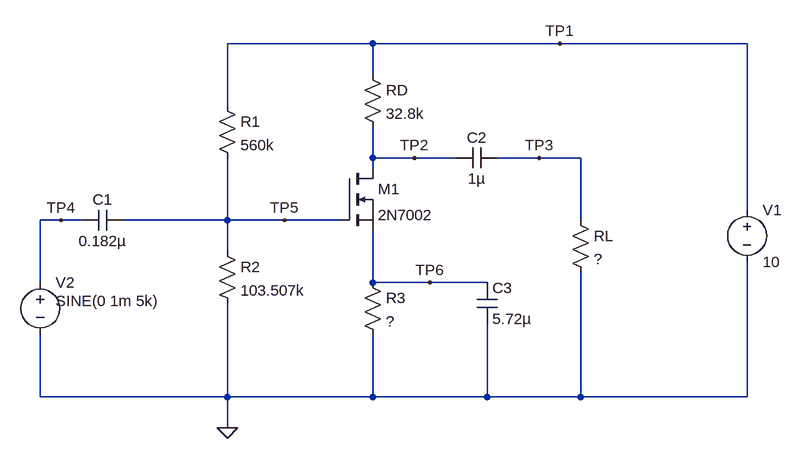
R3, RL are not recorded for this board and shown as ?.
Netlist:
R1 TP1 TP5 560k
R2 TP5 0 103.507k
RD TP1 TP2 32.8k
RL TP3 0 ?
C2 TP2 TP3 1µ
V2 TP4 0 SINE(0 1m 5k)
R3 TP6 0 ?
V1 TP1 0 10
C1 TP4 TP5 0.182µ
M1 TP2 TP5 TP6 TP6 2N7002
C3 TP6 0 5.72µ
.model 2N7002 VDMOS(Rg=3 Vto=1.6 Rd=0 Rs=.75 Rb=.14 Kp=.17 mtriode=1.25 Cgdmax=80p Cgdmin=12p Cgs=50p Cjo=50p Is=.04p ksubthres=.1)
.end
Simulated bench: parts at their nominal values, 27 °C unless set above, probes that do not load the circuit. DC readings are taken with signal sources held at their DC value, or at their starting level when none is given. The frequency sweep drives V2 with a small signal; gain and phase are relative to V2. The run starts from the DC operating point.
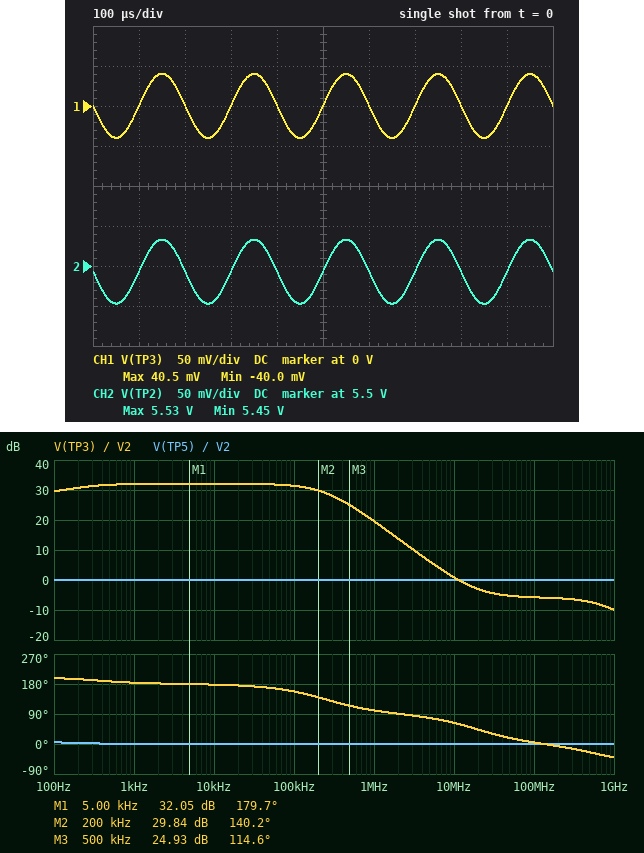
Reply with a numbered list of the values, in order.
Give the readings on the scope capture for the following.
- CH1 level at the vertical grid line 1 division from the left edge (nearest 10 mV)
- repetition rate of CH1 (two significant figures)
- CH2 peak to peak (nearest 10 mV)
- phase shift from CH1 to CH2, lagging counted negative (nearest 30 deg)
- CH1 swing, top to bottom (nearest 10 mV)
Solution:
1. 0 V
2. 5.0 kHz
3. 80 mV
4. 0 deg
5. 80 mV
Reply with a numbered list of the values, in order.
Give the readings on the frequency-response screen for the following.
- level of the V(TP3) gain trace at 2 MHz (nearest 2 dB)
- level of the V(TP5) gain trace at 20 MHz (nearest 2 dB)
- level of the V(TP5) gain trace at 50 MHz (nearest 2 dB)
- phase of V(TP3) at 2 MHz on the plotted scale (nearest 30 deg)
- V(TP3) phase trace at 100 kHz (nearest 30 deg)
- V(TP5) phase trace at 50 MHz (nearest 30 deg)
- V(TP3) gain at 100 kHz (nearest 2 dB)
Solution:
1. 14 dB
2. 0 dB
3. 0 dB
4. 90 deg
5. 150 deg
6. 0 deg
7. 32 dB
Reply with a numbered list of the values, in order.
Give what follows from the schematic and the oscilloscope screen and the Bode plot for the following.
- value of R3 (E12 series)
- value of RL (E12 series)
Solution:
1. 220 Ω
2. 39 kΩ
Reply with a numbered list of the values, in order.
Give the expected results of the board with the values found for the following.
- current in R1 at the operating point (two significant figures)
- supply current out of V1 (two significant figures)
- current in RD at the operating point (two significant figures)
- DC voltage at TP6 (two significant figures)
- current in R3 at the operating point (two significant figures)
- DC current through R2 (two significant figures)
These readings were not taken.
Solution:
1. 15 µA
2. 150 µA
3. 140 µA
4. 30 mV
5. 140 µA
6. 15 µA
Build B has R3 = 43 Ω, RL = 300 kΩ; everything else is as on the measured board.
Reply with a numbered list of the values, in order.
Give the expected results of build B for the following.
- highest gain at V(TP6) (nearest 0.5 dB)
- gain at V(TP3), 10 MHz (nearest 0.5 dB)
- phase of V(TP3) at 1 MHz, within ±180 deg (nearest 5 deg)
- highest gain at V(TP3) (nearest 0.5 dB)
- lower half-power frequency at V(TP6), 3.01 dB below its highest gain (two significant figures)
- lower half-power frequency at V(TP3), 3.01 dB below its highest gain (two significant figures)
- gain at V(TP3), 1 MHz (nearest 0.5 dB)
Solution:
1. -19.0 dB
2. 1.5 dB
3. 95 deg
4. 39.0 dB
5. 9.6 Hz
6. 13 Hz
7. 20.5 dB
